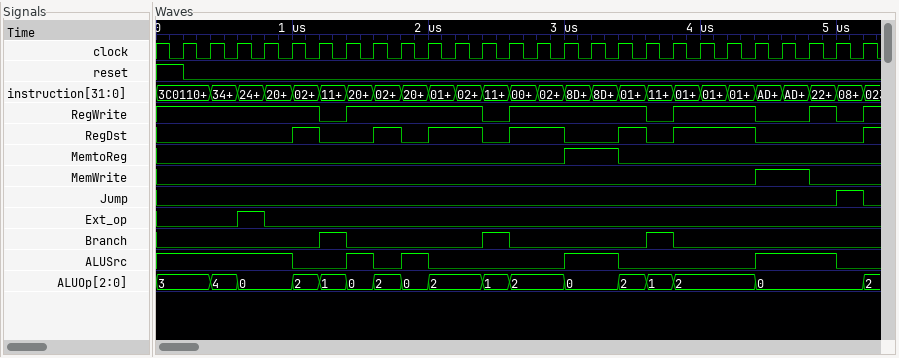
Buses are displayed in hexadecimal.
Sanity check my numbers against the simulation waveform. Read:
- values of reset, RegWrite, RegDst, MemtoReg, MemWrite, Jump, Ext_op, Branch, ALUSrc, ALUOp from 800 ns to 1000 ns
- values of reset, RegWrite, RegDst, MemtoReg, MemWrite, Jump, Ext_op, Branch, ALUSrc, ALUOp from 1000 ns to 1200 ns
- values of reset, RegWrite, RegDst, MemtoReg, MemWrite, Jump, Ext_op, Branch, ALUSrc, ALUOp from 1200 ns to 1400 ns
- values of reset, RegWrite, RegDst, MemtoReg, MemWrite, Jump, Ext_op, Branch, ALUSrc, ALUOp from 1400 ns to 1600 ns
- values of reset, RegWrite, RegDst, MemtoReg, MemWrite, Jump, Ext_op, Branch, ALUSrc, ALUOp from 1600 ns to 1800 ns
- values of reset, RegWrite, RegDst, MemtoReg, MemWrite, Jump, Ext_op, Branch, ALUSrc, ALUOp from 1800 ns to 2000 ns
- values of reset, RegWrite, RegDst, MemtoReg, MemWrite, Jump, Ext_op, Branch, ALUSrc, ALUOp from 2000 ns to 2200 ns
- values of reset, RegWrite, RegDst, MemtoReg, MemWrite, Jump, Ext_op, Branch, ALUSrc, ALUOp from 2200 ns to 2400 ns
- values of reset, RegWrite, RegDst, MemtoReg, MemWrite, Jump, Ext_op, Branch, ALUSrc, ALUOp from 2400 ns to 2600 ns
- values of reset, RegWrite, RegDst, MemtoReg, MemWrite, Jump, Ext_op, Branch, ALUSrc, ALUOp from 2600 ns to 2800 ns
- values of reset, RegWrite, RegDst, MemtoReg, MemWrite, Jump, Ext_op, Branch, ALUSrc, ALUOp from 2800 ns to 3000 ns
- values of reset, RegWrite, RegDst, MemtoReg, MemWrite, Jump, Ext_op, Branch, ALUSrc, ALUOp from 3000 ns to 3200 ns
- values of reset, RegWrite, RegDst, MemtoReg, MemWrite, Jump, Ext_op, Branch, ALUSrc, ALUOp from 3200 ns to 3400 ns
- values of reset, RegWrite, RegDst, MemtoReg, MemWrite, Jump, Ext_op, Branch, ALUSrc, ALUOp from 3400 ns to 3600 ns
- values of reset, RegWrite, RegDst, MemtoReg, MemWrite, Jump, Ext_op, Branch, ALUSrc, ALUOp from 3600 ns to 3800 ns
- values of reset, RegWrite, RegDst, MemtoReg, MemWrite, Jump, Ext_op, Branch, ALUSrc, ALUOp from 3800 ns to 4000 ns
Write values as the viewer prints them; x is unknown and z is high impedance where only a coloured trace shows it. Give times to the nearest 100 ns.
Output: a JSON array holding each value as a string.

["reset=0, RegWrite=1, RegDst=0, MemtoReg=0, MemWrite=0, Jump=0, Ext_op=0, Branch=0, ALUSrc=1, ALUOp=0", "reset=0, RegWrite=1, RegDst=1, MemtoReg=0, MemWrite=0, Jump=0, Ext_op=0, Branch=0, ALUSrc=0, ALUOp=2", "reset=0, RegWrite=0, RegDst=0, MemtoReg=0, MemWrite=0, Jump=0, Ext_op=0, Branch=1, ALUSrc=0, ALUOp=1", "reset=0, RegWrite=1, RegDst=0, MemtoReg=0, MemWrite=0, Jump=0, Ext_op=0, Branch=0, ALUSrc=1, ALUOp=0", "reset=0, RegWrite=1, RegDst=1, MemtoReg=0, MemWrite=0, Jump=0, Ext_op=0, Branch=0, ALUSrc=0, ALUOp=2", "reset=0, RegWrite=1, RegDst=0, MemtoReg=0, MemWrite=0, Jump=0, Ext_op=0, Branch=0, ALUSrc=1, ALUOp=0", "reset=0, RegWrite=1, RegDst=1, MemtoReg=0, MemWrite=0, Jump=0, Ext_op=0, Branch=0, ALUSrc=0, ALUOp=2", "reset=0, RegWrite=1, RegDst=1, MemtoReg=0, MemWrite=0, Jump=0, Ext_op=0, Branch=0, ALUSrc=0, ALUOp=2", "reset=0, RegWrite=0, RegDst=0, MemtoReg=0, MemWrite=0, Jump=0, Ext_op=0, Branch=1, ALUSrc=0, ALUOp=1", "reset=0, RegWrite=1, RegDst=1, MemtoReg=0, MemWrite=0, Jump=0, Ext_op=0, Branch=0, ALUSrc=0, ALUOp=2", "reset=0, RegWrite=1, RegDst=1, MemtoReg=0, MemWrite=0, Jump=0, Ext_op=0, Branch=0, ALUSrc=0, ALUOp=2", "reset=0, RegWrite=1, RegDst=0, MemtoReg=1, MemWrite=0, Jump=0, Ext_op=0, Branch=0, ALUSrc=1, ALUOp=0", "reset=0, RegWrite=1, RegDst=0, MemtoReg=1, MemWrite=0, Jump=0, Ext_op=0, Branch=0, ALUSrc=1, ALUOp=0", "reset=0, RegWrite=1, RegDst=1, MemtoReg=0, MemWrite=0, Jump=0, Ext_op=0, Branch=0, ALUSrc=0, ALUOp=2", "reset=0, RegWrite=0, RegDst=0, MemtoReg=0, MemWrite=0, Jump=0, Ext_op=0, Branch=1, ALUSrc=0, ALUOp=1", "reset=0, RegWrite=1, RegDst=1, MemtoReg=0, MemWrite=0, Jump=0, Ext_op=0, Branch=0, ALUSrc=0, ALUOp=2"]
